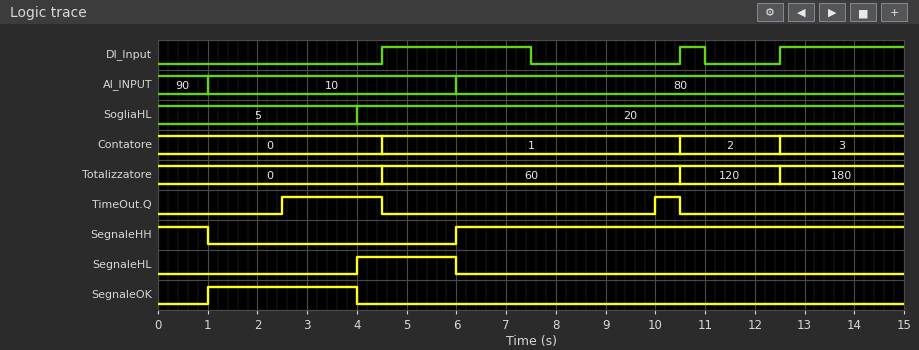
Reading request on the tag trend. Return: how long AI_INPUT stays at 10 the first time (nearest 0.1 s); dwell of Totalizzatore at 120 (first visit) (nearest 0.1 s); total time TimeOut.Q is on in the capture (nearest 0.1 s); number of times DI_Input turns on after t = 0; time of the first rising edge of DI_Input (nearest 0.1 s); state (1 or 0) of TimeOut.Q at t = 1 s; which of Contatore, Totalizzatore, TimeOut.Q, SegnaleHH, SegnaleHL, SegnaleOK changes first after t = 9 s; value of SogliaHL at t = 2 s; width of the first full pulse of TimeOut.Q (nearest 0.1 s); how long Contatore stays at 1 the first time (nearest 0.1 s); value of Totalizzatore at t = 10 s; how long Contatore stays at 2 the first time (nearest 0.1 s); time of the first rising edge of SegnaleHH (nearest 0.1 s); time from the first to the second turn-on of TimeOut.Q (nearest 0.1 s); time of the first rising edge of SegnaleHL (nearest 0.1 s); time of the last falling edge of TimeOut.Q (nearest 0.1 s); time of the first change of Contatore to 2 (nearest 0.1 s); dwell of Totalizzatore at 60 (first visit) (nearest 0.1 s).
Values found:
5.0 s
2.0 s
2.5 s
3
4.5 s
0
TimeOut.Q
5
2.0 s
6.0 s
60
2.0 s
6.0 s
7.5 s
4.0 s
10.5 s
10.5 s
6.0 s
